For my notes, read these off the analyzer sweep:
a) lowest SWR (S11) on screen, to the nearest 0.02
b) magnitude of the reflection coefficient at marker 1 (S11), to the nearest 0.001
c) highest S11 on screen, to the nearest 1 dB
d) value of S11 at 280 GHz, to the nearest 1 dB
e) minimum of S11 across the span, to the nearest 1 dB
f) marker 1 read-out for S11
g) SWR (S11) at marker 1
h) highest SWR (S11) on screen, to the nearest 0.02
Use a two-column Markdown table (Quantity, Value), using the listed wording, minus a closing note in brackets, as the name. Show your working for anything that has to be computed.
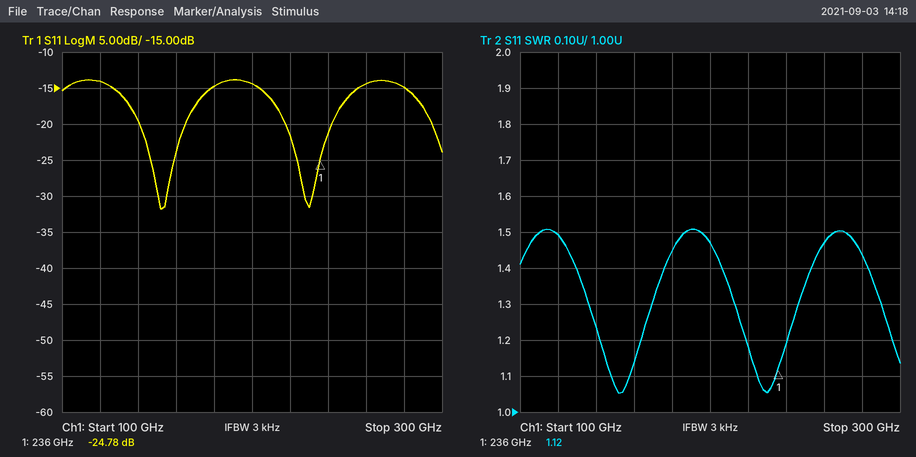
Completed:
| Quantity | Value |
|---|---|
| lowest SWR (S11) on screen, to the nearest 0.02 | 1.06 |
| magnitude of the reflection coefficient at marker 1 (S11), to the nearest 0.001 | 10^(-24.78/20) ≈ 0.058 |
| highest S11 on screen, to the nearest 1 dB | -14 dB |
| value of S11 at 280 GHz, to the nearest 1 dB | -15 dB |
| minimum of S11 across the span, to the nearest 1 dB | -32 dB |
| marker 1 read-out for S11 | -24.78 dB |
| SWR (S11) at marker 1 | 1.12 |
| highest SWR (S11) on screen, to the nearest 0.02 | 1.50 |
